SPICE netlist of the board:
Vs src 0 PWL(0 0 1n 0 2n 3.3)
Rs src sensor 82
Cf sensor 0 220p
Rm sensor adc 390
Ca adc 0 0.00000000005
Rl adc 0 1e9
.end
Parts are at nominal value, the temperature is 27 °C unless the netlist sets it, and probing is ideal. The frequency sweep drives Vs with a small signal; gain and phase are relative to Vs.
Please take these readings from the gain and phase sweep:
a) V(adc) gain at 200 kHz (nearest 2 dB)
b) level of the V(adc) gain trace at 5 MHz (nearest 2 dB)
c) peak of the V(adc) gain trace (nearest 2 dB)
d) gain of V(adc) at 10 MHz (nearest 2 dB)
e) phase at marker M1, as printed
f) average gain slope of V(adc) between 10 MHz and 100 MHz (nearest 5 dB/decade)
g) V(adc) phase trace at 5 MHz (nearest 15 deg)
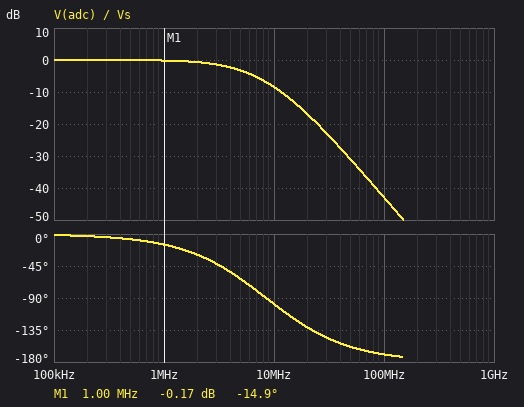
0 dB
-4 dB
0 dB
-8 dB
-14.9 deg
-35 dB/decade
-60 deg
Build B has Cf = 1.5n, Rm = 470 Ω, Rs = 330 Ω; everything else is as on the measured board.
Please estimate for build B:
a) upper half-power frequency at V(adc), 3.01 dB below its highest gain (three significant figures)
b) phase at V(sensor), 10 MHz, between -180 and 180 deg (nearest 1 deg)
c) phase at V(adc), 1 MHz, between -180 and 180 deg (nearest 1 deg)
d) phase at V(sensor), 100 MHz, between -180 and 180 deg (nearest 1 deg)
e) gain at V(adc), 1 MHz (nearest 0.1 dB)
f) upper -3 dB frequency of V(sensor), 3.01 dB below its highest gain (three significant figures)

310 kHz
-87 deg
-81 deg
-90 deg
-10.6 dB
311 kHz
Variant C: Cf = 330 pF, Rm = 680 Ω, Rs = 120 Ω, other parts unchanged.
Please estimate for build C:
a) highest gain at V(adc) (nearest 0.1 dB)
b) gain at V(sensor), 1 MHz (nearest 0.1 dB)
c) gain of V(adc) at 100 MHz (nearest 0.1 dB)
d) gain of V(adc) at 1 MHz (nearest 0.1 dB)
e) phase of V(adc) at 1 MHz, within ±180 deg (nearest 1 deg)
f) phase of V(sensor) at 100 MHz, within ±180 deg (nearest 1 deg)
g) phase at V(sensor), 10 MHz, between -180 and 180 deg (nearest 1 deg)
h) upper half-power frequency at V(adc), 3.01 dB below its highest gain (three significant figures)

0 dB
-0.4 dB
-54.5 dB
-0.6 dB
-28 deg
-87 deg
-66 deg
2.49 MHz
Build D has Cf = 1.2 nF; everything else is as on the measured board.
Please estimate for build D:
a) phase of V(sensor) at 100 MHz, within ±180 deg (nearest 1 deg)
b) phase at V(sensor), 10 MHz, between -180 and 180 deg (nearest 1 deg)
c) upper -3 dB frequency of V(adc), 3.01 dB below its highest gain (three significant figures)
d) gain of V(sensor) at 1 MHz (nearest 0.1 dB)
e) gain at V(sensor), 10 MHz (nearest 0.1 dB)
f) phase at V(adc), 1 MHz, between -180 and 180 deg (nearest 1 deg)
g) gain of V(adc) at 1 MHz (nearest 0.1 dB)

-89 deg
-80 deg
1.49 MHz
-1.5 dB
-16.1 dB
-40 deg
-1.6 dB
